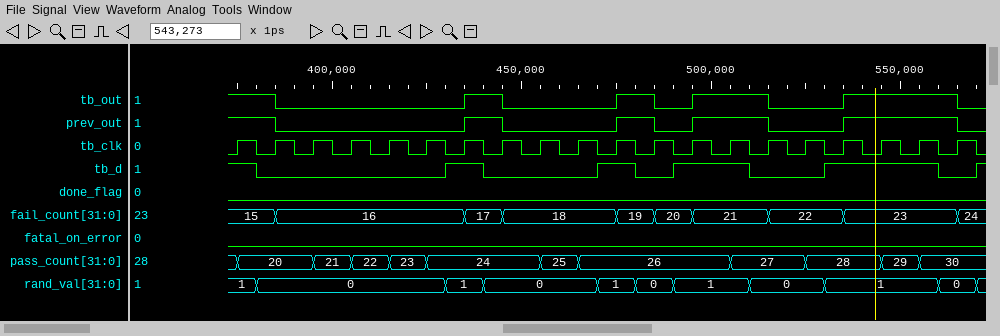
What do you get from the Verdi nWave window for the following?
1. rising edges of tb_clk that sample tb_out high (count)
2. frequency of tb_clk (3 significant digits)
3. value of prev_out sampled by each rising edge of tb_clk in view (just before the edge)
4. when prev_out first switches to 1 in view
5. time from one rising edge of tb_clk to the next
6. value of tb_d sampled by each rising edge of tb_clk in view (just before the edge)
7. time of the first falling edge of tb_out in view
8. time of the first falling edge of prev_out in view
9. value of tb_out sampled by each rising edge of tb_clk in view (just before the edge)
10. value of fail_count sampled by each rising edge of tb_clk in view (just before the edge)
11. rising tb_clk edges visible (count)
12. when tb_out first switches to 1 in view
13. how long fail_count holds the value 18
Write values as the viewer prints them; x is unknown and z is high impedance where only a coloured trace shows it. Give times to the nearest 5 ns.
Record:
9
100 MHz
1 1 0 0 0 0 0 1 0 0 0 1 0 1 1 0 0 1 1 1
435 ns
10 ns
1 0 0 0 0 0 1 0 0 0 1 0 1 1 0 0 1 1 1 0
385 ns
385 ns
1 1 0 0 0 0 0 1 0 0 0 1 0 1 1 0 0 1 1 1
15, 15, 16, 16, 16, 16, 16, 17, 18, 18, 18, 19, 20, 21, 21, 22, 22, 23, 23, 23
20
435 ns
30 ns
